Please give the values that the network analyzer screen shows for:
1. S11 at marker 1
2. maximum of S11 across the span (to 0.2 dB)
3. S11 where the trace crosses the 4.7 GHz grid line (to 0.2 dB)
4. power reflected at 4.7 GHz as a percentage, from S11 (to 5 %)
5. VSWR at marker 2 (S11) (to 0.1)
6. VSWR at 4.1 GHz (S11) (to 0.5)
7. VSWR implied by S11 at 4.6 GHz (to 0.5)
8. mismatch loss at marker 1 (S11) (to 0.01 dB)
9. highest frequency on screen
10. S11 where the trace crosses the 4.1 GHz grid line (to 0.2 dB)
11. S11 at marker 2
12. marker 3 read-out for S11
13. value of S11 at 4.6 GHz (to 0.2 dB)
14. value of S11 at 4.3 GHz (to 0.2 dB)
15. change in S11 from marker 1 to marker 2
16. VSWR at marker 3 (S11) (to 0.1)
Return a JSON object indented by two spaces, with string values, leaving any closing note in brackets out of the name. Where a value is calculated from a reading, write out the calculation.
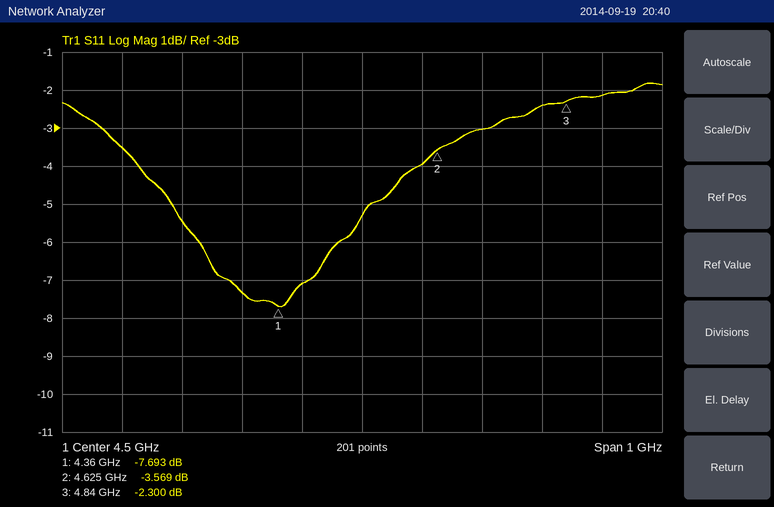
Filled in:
{
  "S11 at marker 1": "-7.693 dB",
  "maximum of S11 across the span": "-1.8 dB",
  "S11 where the trace crosses the 4.7 GHz grid line": "-3.0 dB",
  "power reflected at 4.7 GHz as a percentage, from S11": "10^(-3/10) ≈ 50 %",
  "VSWR at marker 2 (S11)": "(1 + 0.6631)/(1 − 0.6631) ≈ 4.9",
  "VSWR at 4.1 GHz (S11)": "|Γ| = 10^(-3.6/20) = 0.6607; VSWR = (1 + 0.6607)/(1 − 0.6607) ≈ 4.89, so 5.0 to the nearest 0.5",
  "VSWR implied by S11 at 4.6 GHz": "|Γ| = 10^(-4/20) = 0.6310; VSWR = (1 + 0.6310)/(1 − 0.6310) ≈ 4.42, so 4.5 to the nearest 0.5",
  "mismatch loss at marker 1 (S11)": "−10 log10(1 − 10^(-7.693/10)) ≈ 0.81 dB",
  "highest frequency on screen": "5 GHz",
  "S11 where the trace crosses the 4.1 GHz grid line": "-3.6 dB",
  "S11 at marker 2": "-3.569 dB",
  "marker 3 read-out for S11": "-2.300 dB",
  "value of S11 at 4.6 GHz": "-4.0 dB",
  "value of S11 at 4.3 GHz": "-7.4 dB",
  "change in S11 from marker 1 to marker 2": "-3.569 − (-7.693) = 4.124 dB",
  "VSWR at marker 3 (S11)": "(1 + 0.7674)/(1 − 0.7674) ≈ 7.6"
}
